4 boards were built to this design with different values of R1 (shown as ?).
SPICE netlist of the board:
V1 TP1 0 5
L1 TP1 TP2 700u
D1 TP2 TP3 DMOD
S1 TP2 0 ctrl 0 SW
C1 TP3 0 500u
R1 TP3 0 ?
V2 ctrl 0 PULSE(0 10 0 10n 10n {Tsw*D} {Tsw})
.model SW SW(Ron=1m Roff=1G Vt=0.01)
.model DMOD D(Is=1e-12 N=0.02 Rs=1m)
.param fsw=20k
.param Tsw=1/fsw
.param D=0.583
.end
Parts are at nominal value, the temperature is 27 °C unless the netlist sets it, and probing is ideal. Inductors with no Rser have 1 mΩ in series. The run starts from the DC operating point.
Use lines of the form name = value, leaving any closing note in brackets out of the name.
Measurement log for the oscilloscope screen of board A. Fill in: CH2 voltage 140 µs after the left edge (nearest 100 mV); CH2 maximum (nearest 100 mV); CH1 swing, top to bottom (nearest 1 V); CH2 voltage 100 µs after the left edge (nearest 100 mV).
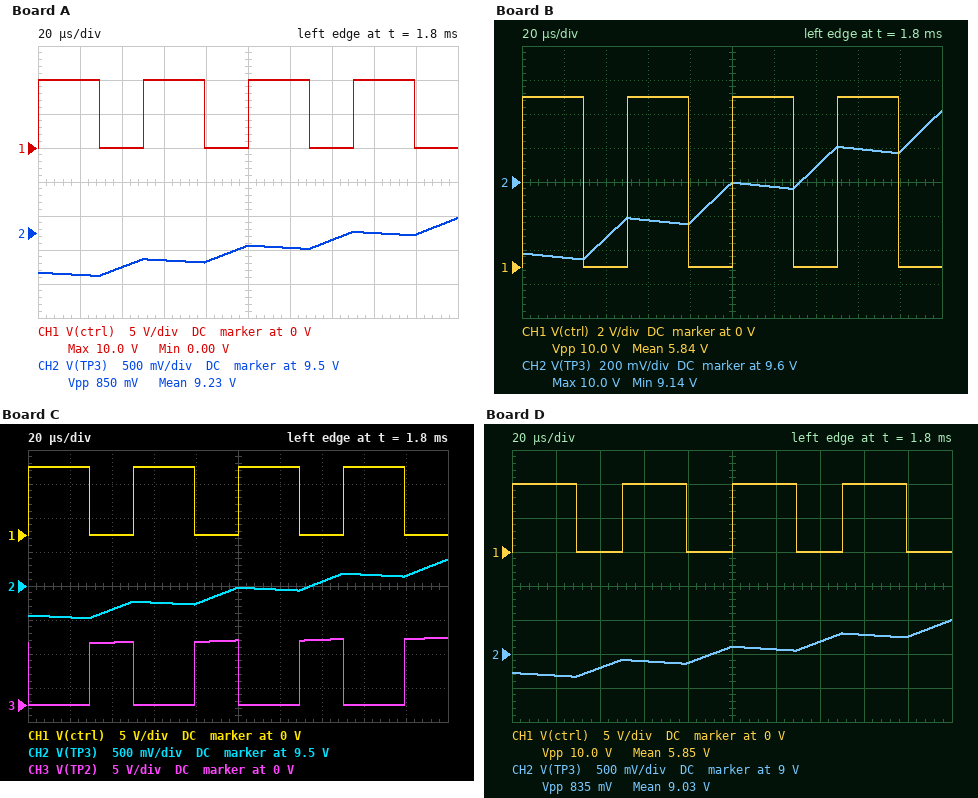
CH2 voltage 140 µs after the left edge = 9.4 V
CH2 maximum = 9.7 V
CH1 swing, top to bottom = 10 V
CH2 voltage 100 µs after the left edge = 9.3 V
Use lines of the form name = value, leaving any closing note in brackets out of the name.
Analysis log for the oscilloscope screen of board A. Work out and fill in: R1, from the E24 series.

R1, from the E24 series = 11 Ω
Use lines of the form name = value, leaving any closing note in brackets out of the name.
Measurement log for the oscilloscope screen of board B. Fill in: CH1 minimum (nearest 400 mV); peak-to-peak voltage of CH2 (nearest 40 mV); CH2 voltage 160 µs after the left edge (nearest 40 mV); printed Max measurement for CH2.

CH1 minimum = 0 V
peak-to-peak voltage of CH2 = 880 mV
CH2 voltage 160 µs after the left edge = 9.80 V
printed Max measurement for CH2 = 10.0 V
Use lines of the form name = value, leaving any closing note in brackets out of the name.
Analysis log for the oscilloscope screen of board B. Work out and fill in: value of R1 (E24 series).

value of R1 = 15 Ω
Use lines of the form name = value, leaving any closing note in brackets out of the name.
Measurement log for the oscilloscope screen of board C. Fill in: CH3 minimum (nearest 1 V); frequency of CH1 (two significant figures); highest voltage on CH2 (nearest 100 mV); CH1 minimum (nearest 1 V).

CH3 minimum = 0 V
frequency of CH1 = 20 kHz
highest voltage on CH2 = 9.9 V
CH1 minimum = 0 V
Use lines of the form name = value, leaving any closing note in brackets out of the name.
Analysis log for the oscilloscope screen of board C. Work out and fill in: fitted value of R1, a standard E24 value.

fitted value of R1, a standard E24 value = 13 Ω
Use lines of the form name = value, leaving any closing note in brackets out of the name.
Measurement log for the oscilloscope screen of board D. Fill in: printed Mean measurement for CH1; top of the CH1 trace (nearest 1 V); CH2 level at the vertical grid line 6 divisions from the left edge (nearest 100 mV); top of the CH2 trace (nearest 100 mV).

printed Mean measurement for CH1 = 5.85 V
top of the CH1 trace = 10 V
CH2 level at the vertical grid line 6 divisions from the left edge = 9.1 V
top of the CH2 trace = 9.5 V
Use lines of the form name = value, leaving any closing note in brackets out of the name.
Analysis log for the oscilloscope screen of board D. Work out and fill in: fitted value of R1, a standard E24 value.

fitted value of R1, a standard E24 value = 9.1 Ω
